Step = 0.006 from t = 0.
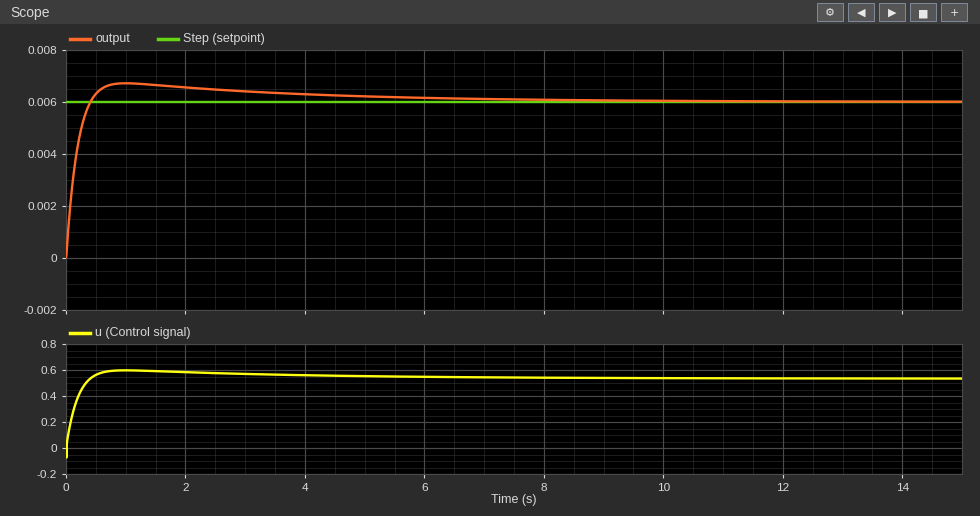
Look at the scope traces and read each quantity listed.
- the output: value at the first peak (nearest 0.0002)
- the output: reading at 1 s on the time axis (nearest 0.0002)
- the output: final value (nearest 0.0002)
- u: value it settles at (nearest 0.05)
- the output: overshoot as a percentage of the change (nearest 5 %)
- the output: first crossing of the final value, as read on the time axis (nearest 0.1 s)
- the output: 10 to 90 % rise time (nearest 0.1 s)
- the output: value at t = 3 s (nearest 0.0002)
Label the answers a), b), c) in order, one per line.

a) 0.0068
b) 0.0068
c) 0.0060
d) 0.55
e) 10 %
f) 0.4 s
g) 0.3 s
h) 0.0064
